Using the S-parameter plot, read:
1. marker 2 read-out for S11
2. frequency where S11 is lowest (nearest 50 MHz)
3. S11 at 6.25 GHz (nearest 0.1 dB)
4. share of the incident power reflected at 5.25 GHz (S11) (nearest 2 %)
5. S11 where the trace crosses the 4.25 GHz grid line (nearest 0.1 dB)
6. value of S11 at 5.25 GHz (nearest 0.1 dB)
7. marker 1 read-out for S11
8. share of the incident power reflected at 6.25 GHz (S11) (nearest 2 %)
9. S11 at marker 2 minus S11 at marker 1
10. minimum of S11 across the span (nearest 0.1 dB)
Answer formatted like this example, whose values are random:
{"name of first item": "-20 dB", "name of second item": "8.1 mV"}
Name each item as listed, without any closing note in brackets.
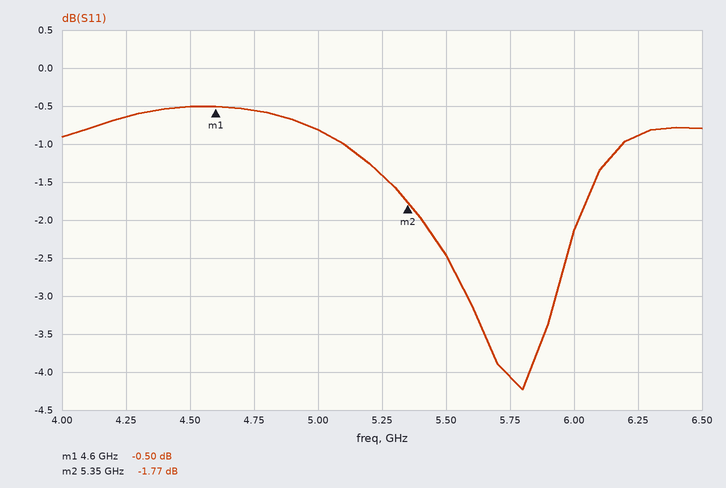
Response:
{"marker 2 read-out for S11": "-1.77 dB", "frequency where S11 is lowest": "5.80 GHz", "S11 at 6.25 GHz": "-0.9 dB", "share of the incident power reflected at 5.25 GHz (S11)": "72 %", "S11 where the trace crosses the 4.25 GHz grid line": "-0.6 dB", "value of S11 at 5.25 GHz": "-1.4 dB", "marker 1 read-out for S11": "-0.50 dB", "share of the incident power reflected at 6.25 GHz (S11)": "82 %", "S11 at marker 2 minus S11 at marker 1": "-1.27 dB", "minimum of S11 across the span": "-4.2 dB"}
